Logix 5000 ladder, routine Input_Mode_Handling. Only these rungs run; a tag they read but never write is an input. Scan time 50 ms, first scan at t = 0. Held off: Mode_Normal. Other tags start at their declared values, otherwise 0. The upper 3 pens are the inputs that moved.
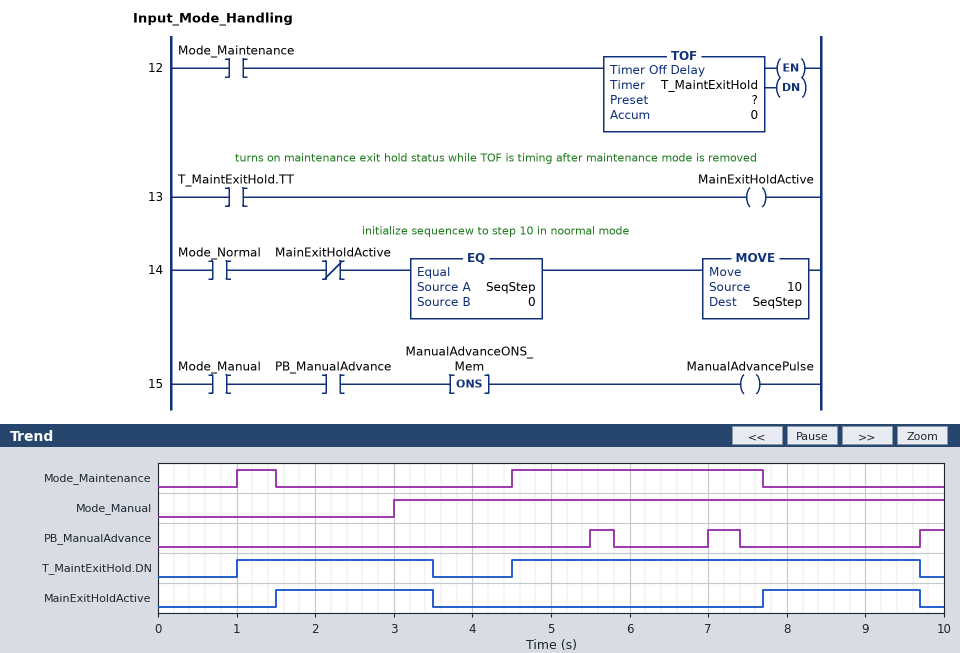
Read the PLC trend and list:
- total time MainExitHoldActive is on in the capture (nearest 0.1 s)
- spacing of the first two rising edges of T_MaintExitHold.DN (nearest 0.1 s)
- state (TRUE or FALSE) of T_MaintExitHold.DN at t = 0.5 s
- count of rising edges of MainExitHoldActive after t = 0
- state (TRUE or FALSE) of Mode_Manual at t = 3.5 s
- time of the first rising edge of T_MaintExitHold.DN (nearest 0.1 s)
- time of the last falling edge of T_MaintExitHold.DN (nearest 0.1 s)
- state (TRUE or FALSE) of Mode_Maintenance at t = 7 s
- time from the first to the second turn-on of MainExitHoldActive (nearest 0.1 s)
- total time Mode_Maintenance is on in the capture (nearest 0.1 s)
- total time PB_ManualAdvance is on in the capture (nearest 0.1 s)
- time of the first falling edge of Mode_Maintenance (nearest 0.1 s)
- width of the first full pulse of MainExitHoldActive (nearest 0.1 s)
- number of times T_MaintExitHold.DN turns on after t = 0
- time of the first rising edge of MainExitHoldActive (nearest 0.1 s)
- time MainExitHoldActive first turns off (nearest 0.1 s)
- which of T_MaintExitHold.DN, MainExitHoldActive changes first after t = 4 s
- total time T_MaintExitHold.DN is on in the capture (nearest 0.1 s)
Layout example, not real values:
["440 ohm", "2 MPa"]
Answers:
["4.0 s", "3.5 s", "FALSE", "2", "TRUE", "1.0 s", "9.7 s", "TRUE", "6.2 s", "3.7 s", "1.0 s", "1.5 s", "2.0 s", "2", "1.5 s", "3.5 s", "T_MaintExitHold.DN", "7.7 s"]
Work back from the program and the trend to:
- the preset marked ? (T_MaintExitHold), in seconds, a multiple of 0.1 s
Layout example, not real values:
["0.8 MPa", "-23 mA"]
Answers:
["2.0 s"]
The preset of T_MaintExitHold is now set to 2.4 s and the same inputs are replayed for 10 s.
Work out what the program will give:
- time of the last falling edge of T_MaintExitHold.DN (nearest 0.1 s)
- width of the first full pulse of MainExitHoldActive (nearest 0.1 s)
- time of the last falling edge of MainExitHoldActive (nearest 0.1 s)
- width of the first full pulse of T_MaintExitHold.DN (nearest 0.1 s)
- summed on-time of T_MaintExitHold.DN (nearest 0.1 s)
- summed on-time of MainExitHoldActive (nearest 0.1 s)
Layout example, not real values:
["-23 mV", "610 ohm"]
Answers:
["3.9 s", "2.4 s", "3.9 s", "2.9 s", "8.4 s", "4.7 s"]
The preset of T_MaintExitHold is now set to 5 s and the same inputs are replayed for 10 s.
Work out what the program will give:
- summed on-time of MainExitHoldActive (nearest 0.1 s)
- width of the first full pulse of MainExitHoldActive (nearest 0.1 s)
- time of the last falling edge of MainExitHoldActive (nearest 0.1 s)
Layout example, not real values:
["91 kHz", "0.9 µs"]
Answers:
["5.3 s", "3.0 s", "4.5 s"]
